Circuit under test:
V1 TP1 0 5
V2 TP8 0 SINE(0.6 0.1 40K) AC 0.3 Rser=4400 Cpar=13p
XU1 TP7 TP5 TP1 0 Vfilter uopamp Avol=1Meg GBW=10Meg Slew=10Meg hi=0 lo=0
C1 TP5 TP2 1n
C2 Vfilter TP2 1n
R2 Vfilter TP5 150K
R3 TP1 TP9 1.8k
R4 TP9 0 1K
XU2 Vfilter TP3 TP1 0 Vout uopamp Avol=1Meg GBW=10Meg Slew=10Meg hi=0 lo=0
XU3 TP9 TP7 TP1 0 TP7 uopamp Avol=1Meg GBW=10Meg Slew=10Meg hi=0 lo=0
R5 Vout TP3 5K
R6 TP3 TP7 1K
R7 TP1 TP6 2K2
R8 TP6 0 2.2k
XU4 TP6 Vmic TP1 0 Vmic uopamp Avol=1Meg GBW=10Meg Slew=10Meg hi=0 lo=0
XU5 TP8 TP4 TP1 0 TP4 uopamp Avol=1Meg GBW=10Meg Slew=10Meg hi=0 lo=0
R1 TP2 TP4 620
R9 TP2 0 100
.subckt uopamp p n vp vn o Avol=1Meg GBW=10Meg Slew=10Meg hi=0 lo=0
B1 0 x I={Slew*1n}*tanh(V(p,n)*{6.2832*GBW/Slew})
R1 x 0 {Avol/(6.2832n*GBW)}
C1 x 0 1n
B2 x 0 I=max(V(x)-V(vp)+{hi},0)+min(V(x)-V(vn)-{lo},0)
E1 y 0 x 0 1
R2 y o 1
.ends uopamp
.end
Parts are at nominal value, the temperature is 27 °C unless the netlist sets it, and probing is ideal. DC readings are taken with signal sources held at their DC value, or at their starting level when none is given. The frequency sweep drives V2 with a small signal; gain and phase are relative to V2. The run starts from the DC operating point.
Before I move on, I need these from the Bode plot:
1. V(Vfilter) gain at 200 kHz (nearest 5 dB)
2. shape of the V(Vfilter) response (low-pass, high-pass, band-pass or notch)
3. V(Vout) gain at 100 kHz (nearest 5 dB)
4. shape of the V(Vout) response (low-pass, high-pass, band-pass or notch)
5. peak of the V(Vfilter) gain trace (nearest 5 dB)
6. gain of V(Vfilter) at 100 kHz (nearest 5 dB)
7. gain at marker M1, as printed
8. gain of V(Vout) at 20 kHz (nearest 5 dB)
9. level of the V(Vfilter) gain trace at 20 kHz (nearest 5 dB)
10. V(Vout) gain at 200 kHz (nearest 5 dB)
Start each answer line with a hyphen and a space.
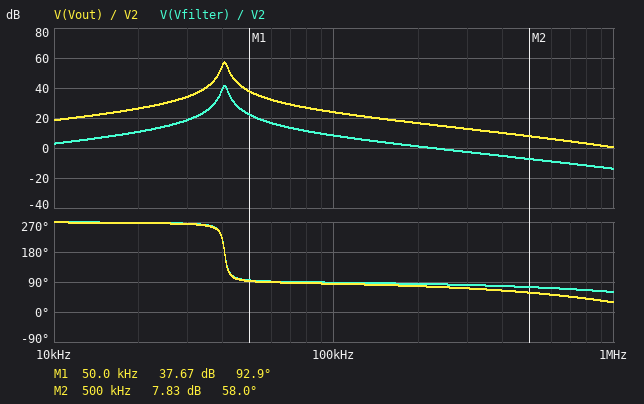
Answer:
- 0 dB
- band-pass
- 25 dB
- band-pass
- 40 dB
- 10 dB
- 37.67 dB
- 25 dB
- 10 dB
- 15 dB
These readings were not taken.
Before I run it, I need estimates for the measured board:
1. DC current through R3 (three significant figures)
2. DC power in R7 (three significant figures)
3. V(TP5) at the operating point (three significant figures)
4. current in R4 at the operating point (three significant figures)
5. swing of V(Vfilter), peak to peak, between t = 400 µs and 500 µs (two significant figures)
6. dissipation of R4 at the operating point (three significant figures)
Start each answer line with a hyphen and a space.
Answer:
- 1.79 mA
- 2.84 mW
- 1.79 V
- 1.79 mA
- 4.2 V
- 3.19 mW
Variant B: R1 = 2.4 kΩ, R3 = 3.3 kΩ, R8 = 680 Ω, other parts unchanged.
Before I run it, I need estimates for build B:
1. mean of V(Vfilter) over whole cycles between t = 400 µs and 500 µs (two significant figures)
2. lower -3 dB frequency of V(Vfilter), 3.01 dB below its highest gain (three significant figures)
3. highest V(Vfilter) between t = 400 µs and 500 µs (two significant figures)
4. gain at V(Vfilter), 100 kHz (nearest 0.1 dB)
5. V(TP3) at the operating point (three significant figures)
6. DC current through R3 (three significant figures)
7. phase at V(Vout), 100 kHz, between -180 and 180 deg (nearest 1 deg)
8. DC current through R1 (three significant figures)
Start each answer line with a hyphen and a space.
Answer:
- 1.2 V
- 37.9 kHz
- 2.4 V
- -3.5 dB
- 1.16 V
- 1.16 mA
- 85 deg
- 240 µA
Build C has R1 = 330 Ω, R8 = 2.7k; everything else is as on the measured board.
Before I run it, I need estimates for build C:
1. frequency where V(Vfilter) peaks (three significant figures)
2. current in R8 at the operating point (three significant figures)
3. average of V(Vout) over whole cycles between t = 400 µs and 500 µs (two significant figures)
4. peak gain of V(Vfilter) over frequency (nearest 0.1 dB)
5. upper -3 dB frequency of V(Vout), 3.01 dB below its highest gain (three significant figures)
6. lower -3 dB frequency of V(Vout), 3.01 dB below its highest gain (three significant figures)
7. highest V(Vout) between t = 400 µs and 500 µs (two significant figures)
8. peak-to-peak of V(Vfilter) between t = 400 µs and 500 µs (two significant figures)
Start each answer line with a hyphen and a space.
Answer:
- 42.7 kHz
- 1.02 mA
- 2.2 V
- 47.0 dB
- 43.6 kHz
- 41.8 kHz
- 5.0 V
- 4.6 V
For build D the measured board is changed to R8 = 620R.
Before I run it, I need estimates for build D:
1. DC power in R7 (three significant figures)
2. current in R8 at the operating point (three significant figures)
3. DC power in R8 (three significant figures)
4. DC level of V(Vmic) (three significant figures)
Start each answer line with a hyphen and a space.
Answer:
- 6.92 mW
- 1.77 mA
- 1.95 mW
- 1.10 V
